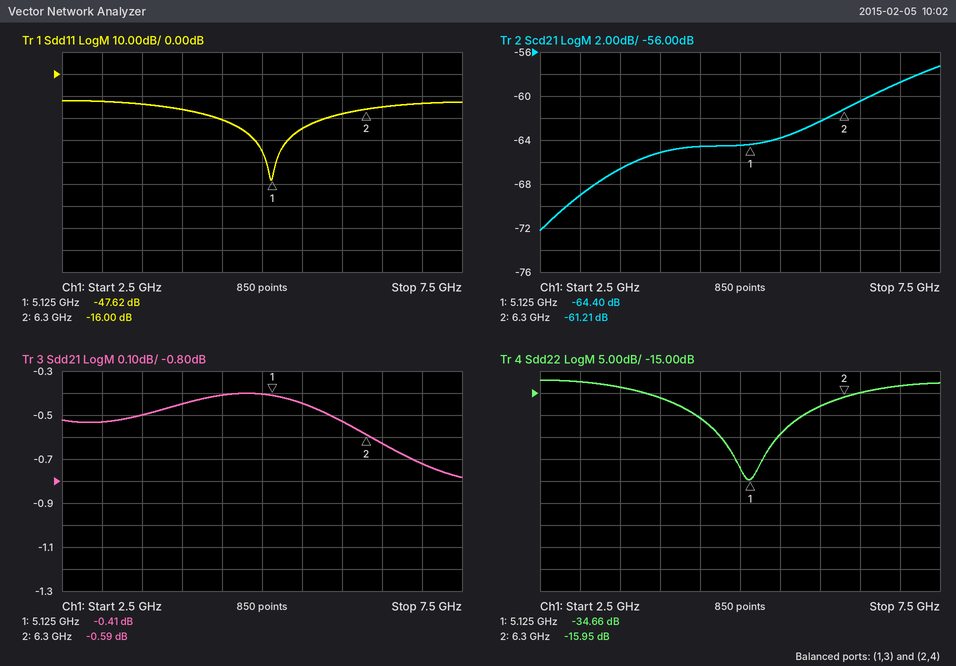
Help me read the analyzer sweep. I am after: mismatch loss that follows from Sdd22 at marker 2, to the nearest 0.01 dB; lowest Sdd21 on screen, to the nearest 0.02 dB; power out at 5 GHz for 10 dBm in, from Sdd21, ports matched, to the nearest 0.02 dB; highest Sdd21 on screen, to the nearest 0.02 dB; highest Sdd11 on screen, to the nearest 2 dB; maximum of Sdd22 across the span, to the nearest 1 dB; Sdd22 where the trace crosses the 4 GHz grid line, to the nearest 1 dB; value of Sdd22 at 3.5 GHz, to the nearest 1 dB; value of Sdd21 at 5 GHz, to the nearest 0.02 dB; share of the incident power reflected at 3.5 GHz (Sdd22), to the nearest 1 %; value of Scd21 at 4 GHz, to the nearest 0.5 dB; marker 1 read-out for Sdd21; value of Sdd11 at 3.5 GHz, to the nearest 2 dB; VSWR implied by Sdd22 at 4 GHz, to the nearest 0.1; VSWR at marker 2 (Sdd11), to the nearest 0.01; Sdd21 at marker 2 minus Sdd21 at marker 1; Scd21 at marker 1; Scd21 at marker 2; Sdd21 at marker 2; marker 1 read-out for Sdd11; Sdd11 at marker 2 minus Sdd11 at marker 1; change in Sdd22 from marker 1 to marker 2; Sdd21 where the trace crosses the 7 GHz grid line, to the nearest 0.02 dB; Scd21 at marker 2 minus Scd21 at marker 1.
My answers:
0.11 dB
-0.78 dB
9.60 dBm
-0.40 dB
-12 dB
-12 dB
-16 dB
-14 dB
-0.40 dB
4 %
-65.0 dB
-0.41 dB
-14 dB
1.4
1.38
-0.18 dB
-64.40 dB
-61.21 dB
-0.59 dB
-47.62 dB
31.62 dB
18.71 dB
-0.72 dB
3.19 dB
